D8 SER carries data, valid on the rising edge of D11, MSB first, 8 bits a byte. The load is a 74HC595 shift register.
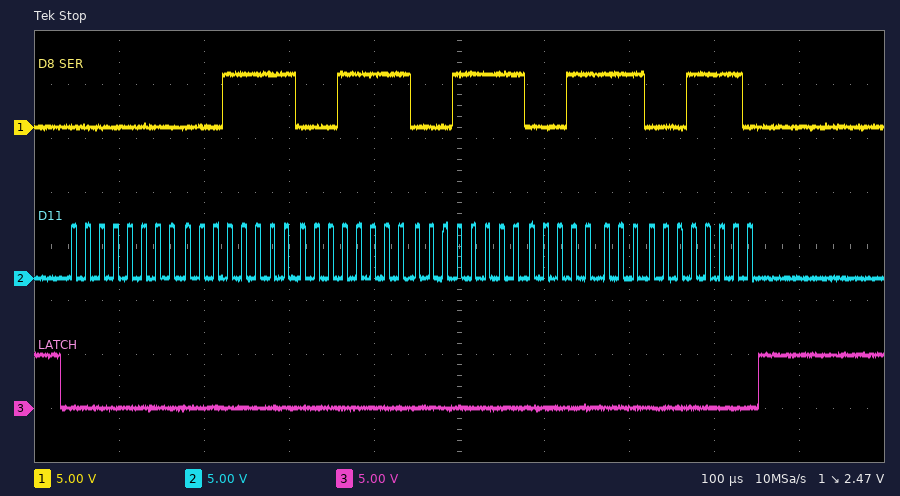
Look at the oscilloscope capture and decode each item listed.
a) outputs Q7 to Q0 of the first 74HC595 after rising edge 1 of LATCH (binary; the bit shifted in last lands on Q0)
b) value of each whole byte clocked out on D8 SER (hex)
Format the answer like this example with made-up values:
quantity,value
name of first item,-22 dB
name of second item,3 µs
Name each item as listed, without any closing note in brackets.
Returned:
quantity,value
outputs Q7 to Q0 of the first 74HC595 after rising edge 1 of LATCH,00011110
value of each whole byte clocked out on D8 SER,0x00 0x1F 0x1F 0x1F 0x1F 0x1E
